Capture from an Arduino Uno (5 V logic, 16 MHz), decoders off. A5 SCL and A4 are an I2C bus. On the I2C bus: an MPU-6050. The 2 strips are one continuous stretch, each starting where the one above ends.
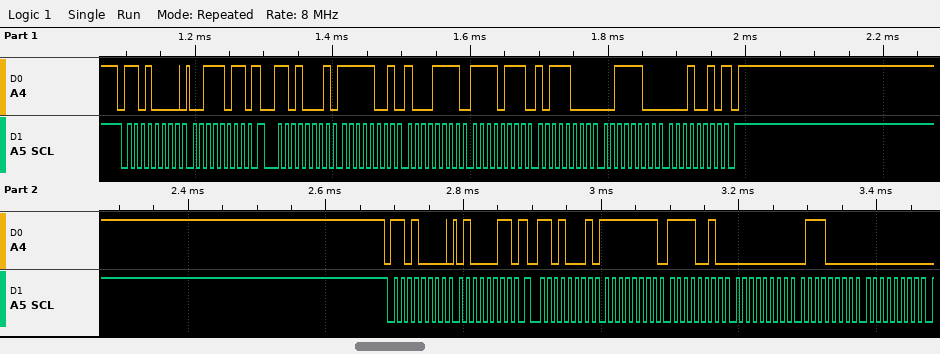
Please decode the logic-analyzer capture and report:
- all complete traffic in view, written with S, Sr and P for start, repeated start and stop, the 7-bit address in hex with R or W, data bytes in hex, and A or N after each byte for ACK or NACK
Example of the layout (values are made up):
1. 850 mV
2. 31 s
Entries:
1. S 68W A 3B A Sr 68R A F9 A 8F A F7 A B8 A 3C A 12 N P S 68W A 43 A Sr 68R A FF A F2 A 00 A 70 A 00 A
